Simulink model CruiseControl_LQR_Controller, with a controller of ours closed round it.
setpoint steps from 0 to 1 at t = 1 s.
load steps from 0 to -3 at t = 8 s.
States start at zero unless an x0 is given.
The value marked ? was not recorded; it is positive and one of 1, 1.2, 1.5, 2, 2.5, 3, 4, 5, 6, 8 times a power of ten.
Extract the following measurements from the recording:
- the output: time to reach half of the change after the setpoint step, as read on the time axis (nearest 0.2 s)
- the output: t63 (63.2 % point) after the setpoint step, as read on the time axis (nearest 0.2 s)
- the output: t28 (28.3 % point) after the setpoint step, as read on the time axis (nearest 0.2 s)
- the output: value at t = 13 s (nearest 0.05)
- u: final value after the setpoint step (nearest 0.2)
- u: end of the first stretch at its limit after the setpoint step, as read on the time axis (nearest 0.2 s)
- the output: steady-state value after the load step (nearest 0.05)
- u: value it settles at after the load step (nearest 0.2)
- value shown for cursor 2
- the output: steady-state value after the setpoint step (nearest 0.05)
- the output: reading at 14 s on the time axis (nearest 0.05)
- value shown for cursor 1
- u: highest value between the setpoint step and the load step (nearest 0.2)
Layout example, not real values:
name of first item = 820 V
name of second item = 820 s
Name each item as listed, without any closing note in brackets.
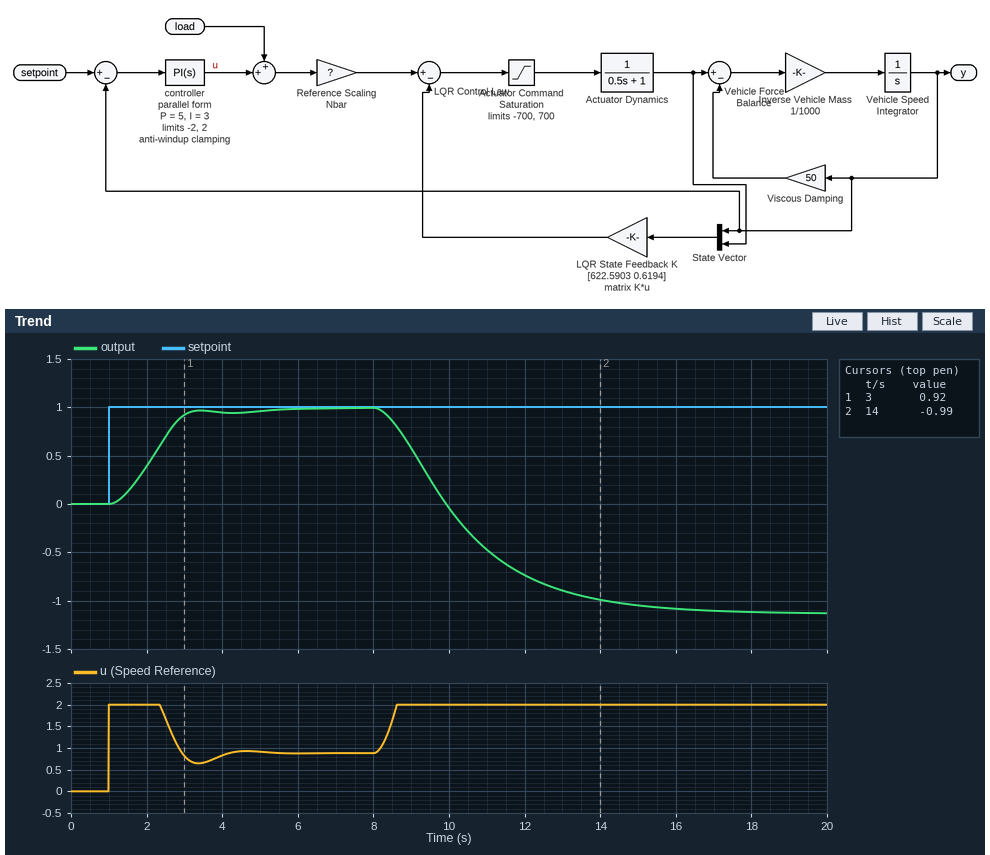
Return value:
the output: time to reach half of the change after the setpoint step, as read on the time axis = 2.2 s
the output: t63 (63.2 % point) after the setpoint step, as read on the time axis = 2.4 s
the output: t28 (28.3 % point) after the setpoint step, as read on the time axis = 1.8 s
the output: value at t = 13 s = -0.90
u: final value after the setpoint step = 0.8
u: end of the first stretch at its limit after the setpoint step, as read on the time axis = 2.4 s
the output: steady-state value after the load step = -1.15
u: value it settles at after the load step = 2.0
value shown for cursor 2 = -0.99
the output: steady-state value after the setpoint step = 1.00
the output: reading at 14 s on the time axis = -1.00
value shown for cursor 1 = 0.92
u: highest value between the setpoint step and the load step = 2.0
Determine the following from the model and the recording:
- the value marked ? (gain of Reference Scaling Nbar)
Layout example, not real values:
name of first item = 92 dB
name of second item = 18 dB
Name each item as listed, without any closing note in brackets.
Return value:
the value marked ? = 800
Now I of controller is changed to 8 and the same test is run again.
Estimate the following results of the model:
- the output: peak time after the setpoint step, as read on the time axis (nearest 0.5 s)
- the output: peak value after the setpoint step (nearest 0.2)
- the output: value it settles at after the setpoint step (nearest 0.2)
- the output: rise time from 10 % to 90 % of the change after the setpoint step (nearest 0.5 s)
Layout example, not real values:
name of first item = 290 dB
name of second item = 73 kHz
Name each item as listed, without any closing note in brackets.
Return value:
the output: peak time after the setpoint step, as read on the time axis = 3.5 s
the output: peak value after the setpoint step = 1.0
the output: value it settles at after the setpoint step = 1.0
the output: rise time from 10 % to 90 % of the change after the setpoint step = 1.5 s
